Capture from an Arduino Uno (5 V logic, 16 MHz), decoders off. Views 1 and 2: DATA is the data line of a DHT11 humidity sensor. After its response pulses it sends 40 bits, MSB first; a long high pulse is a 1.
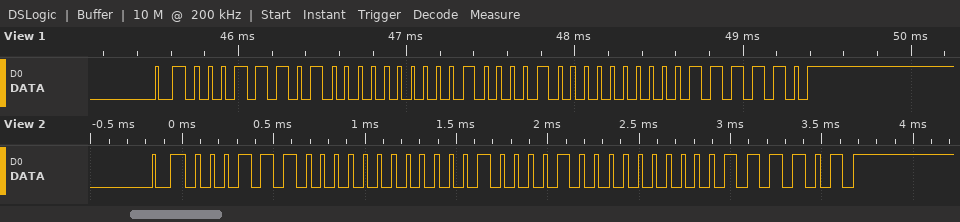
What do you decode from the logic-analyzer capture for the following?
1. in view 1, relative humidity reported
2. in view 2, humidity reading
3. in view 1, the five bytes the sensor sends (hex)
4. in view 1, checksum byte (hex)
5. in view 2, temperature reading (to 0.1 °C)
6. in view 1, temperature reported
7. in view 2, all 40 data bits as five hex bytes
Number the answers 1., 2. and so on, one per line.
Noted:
1. 29 %
2. 28 %
3. 1D 00 21 00 3E
4. 0x3E
5. 33.0 °C
6. 33.0 °C
7. 1C 00 21 00 3D
